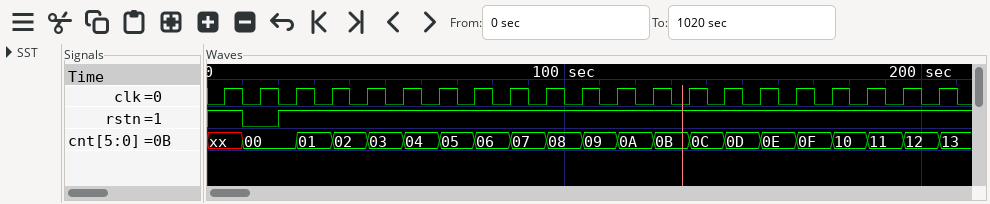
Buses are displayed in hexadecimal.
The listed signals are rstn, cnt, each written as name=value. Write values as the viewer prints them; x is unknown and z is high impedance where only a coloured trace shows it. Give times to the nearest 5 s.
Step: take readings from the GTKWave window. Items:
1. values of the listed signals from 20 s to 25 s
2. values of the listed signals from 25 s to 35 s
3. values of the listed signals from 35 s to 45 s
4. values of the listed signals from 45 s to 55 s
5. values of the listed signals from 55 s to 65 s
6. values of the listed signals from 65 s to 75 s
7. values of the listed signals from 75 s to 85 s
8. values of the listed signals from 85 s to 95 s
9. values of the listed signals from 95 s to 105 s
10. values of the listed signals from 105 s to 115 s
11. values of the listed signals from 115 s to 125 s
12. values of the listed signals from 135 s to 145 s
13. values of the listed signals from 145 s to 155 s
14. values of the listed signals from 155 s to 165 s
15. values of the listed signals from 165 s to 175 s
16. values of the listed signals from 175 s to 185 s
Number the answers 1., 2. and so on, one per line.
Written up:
1. rstn=1, cnt=00
2. rstn=1, cnt=01
3. rstn=1, cnt=02
4. rstn=1, cnt=03
5. rstn=1, cnt=04
6. rstn=1, cnt=05
7. rstn=1, cnt=06
8. rstn=1, cnt=07
9. rstn=1, cnt=08
10. rstn=1, cnt=09
11. rstn=1, cnt=0A
12. rstn=1, cnt=0C
13. rstn=1, cnt=0D
14. rstn=1, cnt=0E
15. rstn=1, cnt=0F
16. rstn=1, cnt=10
